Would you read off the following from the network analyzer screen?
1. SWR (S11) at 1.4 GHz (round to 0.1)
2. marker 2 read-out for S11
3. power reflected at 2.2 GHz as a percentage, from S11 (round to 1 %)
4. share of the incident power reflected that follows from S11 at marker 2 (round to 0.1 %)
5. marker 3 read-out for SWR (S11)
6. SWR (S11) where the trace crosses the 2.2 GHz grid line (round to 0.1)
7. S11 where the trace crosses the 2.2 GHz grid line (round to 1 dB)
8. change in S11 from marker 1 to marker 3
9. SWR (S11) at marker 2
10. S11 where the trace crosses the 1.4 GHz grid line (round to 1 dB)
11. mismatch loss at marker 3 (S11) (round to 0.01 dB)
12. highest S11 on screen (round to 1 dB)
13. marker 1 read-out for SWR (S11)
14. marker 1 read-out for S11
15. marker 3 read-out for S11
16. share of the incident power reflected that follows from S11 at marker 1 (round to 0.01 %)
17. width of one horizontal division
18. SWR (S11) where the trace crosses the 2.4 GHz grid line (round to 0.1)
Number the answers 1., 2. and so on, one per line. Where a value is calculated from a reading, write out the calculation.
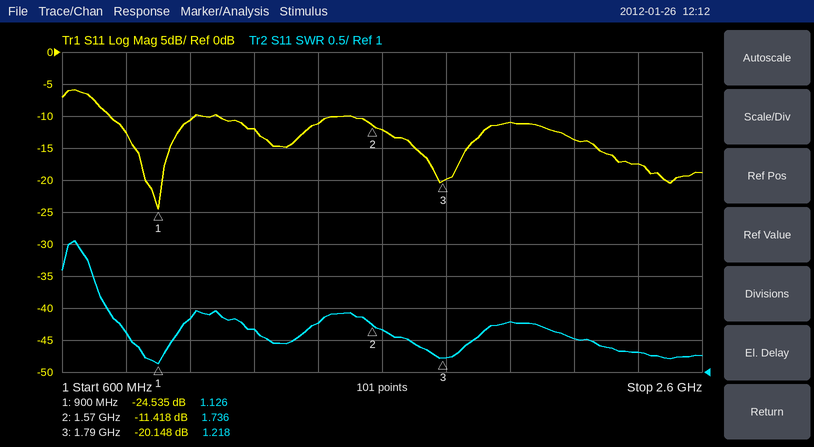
1. 1.8
2. -11.418 dB
3. 10^(-14/10) ≈ 4 %
4. 10^(-11.418/10) ≈ 7.2 %
5. 1.218
6. 1.5
7. -14 dB
8. -20.148 − (-24.535) = 4.387 dB
9. 1.736
10. -11 dB
11. −10 log10(1 − 10^(-20.148/10)) ≈ 0.04 dB
12. -6 dB
13. 1.126
14. -24.535 dB
15. -20.148 dB
16. 10^(-24.535/10) ≈ 0.35 %
17. 200 MHz
18. 1.3
